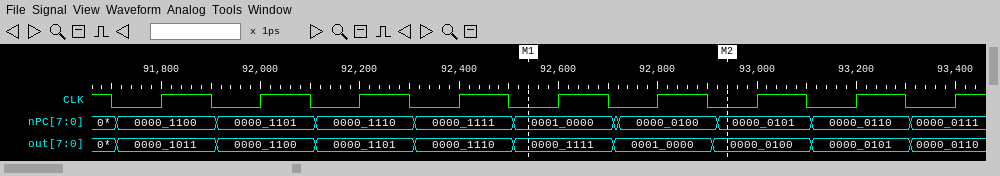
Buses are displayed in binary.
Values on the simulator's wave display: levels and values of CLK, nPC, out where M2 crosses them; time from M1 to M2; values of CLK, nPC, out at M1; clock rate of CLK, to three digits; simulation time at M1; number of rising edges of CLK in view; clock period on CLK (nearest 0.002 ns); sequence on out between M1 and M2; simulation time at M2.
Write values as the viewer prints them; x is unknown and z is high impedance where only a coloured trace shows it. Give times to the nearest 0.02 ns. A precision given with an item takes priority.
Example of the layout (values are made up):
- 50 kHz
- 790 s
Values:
- CLK=0, nPC=0000_0101, out=0000_0100
- 0.4 ns
- CLK=0, nPC=0001_0000, out=0000_1111
- 5.00 GHz
- 92.54 ns
- 9
- 0.2 ns
- 0000_1111, 0001_0000, 0000_0100
- 92.94 ns
